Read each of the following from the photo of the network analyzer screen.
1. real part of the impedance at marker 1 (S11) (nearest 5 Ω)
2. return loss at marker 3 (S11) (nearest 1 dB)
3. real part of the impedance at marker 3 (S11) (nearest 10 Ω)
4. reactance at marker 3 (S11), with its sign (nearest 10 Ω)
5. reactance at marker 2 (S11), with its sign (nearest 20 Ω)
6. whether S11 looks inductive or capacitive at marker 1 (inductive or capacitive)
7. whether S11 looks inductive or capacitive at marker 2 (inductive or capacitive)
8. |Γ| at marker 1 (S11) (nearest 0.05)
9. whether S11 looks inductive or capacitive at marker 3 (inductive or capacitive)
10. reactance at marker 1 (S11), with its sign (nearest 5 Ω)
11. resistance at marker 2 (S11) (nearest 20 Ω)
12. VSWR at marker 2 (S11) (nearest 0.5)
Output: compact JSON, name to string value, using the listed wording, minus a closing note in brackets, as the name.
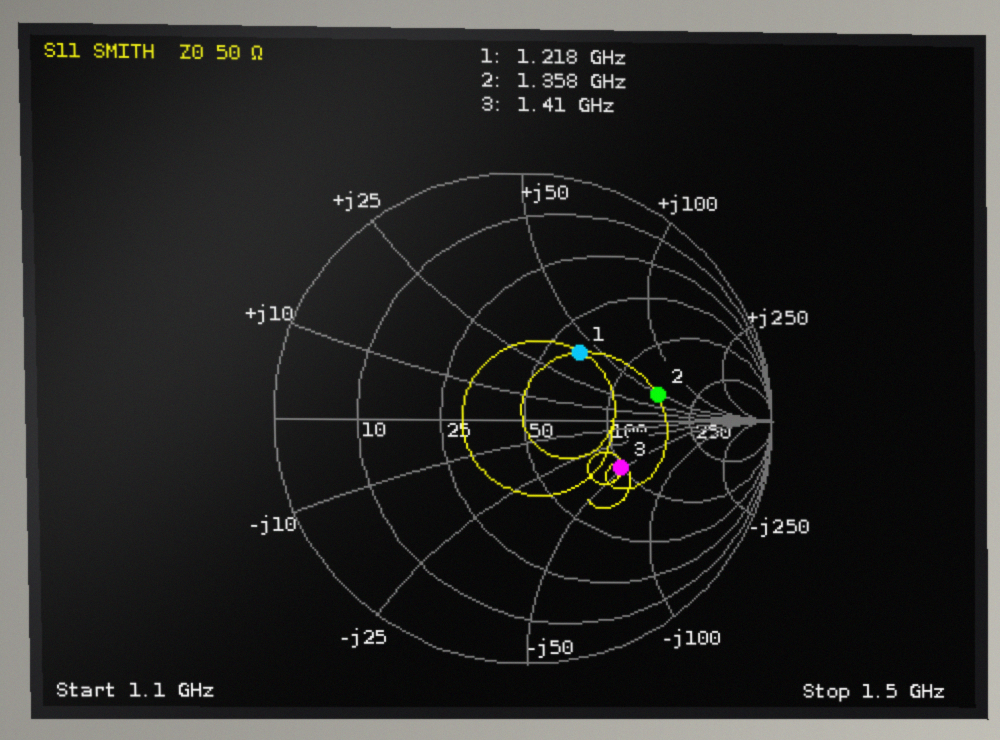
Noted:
{"real part of the impedance at marker 1 (S11)": "65 Ω", "return loss at marker 3 (S11)": "7 dB", "real part of the impedance at marker 3 (S11)": "100 Ω", "reactance at marker 3 (S11), with its sign": "-50 Ω", "reactance at marker 2 (S11), with its sign": "+40 Ω", "whether S11 looks inductive or capacitive at marker 1": "inductive", "whether S11 looks inductive or capacitive at marker 2": "inductive", "|Γ| at marker 1 (S11)": "0.35", "whether S11 looks inductive or capacitive at marker 3": "capacitive", "reactance at marker 1 (S11), with its sign": "+40 Ω", "resistance at marker 2 (S11)": "160 Ω", "VSWR at marker 2 (S11)": "3.5"}
